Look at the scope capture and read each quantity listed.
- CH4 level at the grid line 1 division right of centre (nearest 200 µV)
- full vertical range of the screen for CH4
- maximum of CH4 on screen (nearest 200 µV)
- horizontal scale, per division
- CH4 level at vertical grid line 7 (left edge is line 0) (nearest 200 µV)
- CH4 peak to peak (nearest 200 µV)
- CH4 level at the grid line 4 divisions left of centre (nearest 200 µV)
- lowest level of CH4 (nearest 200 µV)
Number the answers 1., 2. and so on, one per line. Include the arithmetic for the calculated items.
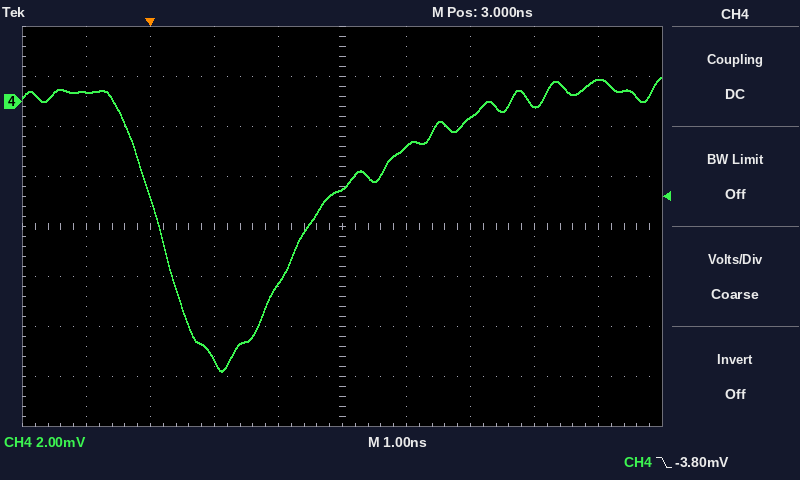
1. -1.8 mV
2. 16 mV
3. 1.0 mV
4. 1 ns
5. -600 µV
6. 1.0 mV − (-10.8 mV) = 11.8 mV
7. 400 µV
8. -10.8 mV
